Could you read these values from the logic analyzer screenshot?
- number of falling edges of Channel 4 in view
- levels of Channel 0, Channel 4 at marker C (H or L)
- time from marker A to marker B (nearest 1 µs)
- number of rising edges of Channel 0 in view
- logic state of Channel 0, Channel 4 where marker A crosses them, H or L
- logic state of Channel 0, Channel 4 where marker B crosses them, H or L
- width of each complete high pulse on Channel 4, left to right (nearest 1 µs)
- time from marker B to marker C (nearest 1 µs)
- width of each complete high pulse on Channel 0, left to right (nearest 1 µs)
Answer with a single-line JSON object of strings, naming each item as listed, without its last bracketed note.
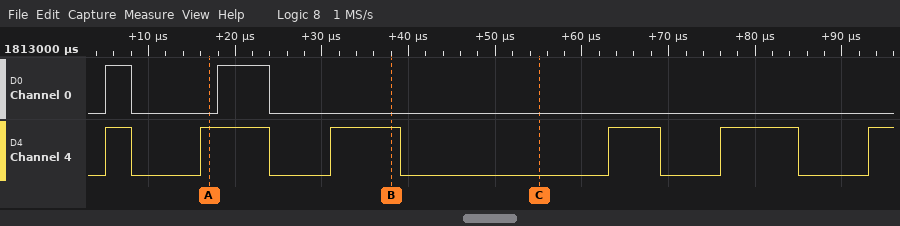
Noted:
{"number of falling edges of Channel 4 in view": "5", "levels of Channel 0, Channel 4 at marker C": "Channel 0=L, Channel 4=L", "time from marker A to marker B": "21 µs", "number of rising edges of Channel 0 in view": "2", "logic state of Channel 0, Channel 4 where marker A crosses them, H or L": "Channel 0=L, Channel 4=H", "logic state of Channel 0, Channel 4 where marker B crosses them, H or L": "Channel 0=L, Channel 4=H", "width of each complete high pulse on Channel 4, left to right": "3 µs, 8 µs, 8 µs, 6 µs, 9 µs", "time from marker B to marker C": "17 µs", "width of each complete high pulse on Channel 0, left to right": "3 µs, 6 µs"}
